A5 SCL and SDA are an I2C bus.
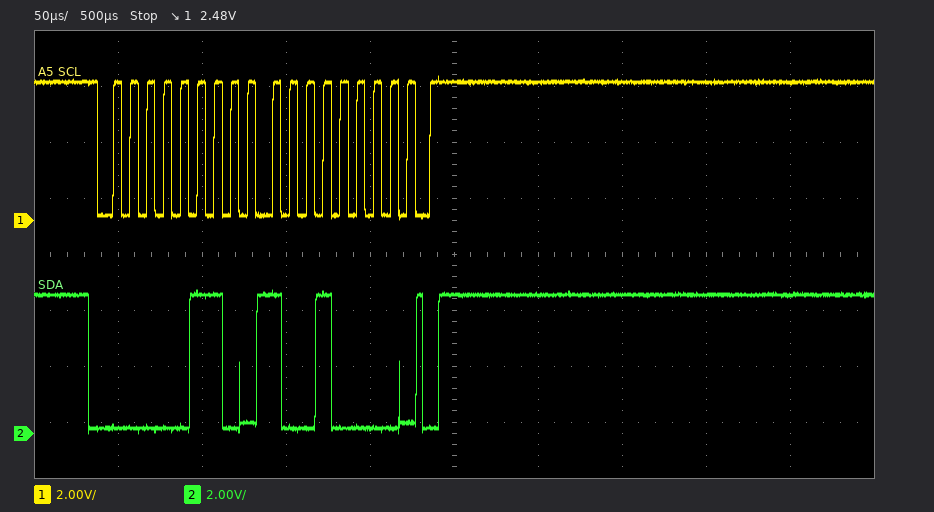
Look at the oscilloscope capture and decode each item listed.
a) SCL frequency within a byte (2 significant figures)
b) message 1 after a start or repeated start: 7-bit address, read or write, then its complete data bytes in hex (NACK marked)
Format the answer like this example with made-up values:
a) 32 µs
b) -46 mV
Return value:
a) 100 kHz
b) 0x03 write: 90
